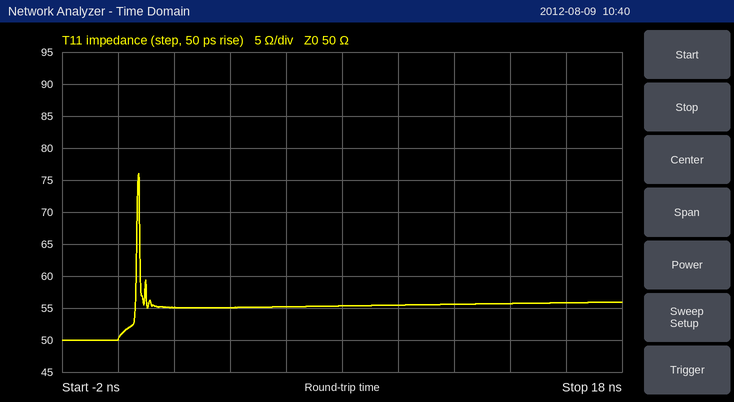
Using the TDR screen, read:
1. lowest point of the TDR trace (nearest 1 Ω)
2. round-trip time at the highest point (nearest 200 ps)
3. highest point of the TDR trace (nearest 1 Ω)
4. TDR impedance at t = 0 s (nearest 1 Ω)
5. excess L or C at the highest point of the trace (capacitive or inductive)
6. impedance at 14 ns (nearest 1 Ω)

50 Ω
800 ps
76 Ω
50 Ω
inductive
56 Ω
